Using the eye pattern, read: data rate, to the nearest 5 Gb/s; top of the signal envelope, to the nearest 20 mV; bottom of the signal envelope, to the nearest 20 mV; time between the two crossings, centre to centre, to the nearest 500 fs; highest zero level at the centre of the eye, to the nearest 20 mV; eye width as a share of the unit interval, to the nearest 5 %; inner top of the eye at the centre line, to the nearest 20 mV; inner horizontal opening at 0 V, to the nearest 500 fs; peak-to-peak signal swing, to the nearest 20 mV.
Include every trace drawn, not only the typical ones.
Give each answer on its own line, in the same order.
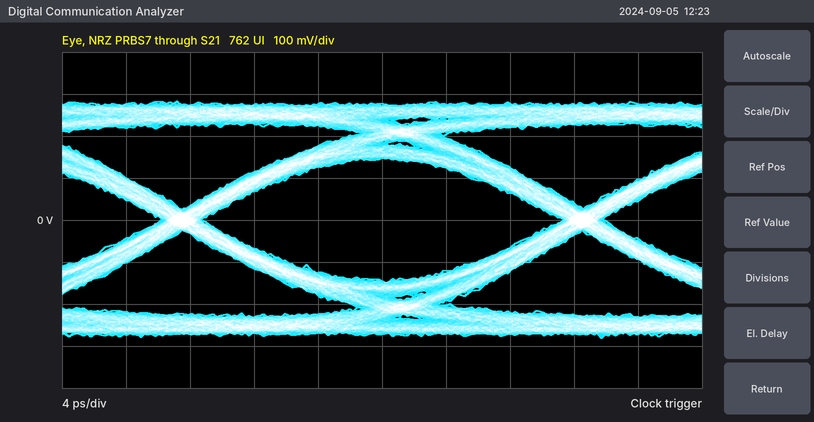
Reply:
40 Gb/s
280 mV
-280 mV
25.0 ps
-140 mV
90 %
140 mV
22.5 ps
560 mV
